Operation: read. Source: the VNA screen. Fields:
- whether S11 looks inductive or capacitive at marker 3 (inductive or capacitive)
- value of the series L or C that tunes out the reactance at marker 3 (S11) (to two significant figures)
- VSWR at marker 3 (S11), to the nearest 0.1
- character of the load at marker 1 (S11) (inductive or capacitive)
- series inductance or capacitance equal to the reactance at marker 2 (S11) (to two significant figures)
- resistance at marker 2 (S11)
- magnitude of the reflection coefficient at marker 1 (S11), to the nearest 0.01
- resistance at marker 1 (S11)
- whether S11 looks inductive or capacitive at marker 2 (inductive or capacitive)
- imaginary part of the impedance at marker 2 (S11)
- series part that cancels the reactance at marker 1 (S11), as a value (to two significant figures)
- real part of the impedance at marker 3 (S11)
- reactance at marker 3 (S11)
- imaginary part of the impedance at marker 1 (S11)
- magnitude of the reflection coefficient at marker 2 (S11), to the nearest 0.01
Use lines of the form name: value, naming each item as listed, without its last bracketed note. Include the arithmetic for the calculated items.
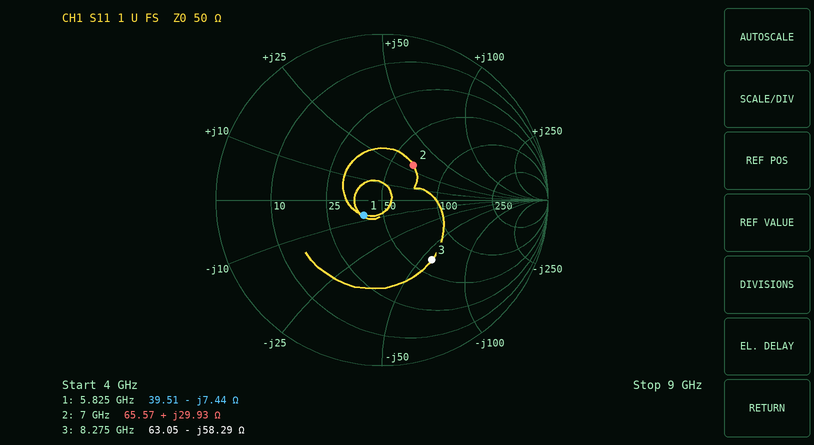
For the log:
whether S11 looks inductive or capacitive at marker 3: capacitive
value of the series L or C that tunes out the reactance at marker 3 (S11): L = 58.29 Ω/(2π × 8.275 GHz) ≈ 1.1 nH
VSWR at marker 3 (S11), to the nearest 0.1: 2.8
character of the load at marker 1 (S11): capacitive
series inductance or capacitance equal to the reactance at marker 2 (S11): L = 29.93 Ω/(2π × 7 GHz) ≈ 681 pH, so 680 pH to two significant figures
resistance at marker 2: 65.57 Ω
magnitude of the reflection coefficient at marker 1 (S11), to the nearest 0.01: 0.14
resistance at marker 1: 39.51 Ω
whether S11 looks inductive or capacitive at marker 2: inductive
imaginary part of the impedance at marker 2: +29.93 Ω
series part that cancels the reactance at marker 1 (S11), as a value: L = 7.44 Ω/(2π × 5.825 GHz) ≈ 203 pH, so 200 pH to two significant figures
real part of the impedance at marker 3: 63.05 Ω
reactance at marker 3: -58.29 Ω
imaginary part of the impedance at marker 1: -7.44 Ω
magnitude of the reflection coefficient at marker 2 (S11), to the nearest 0.01: 0.28
